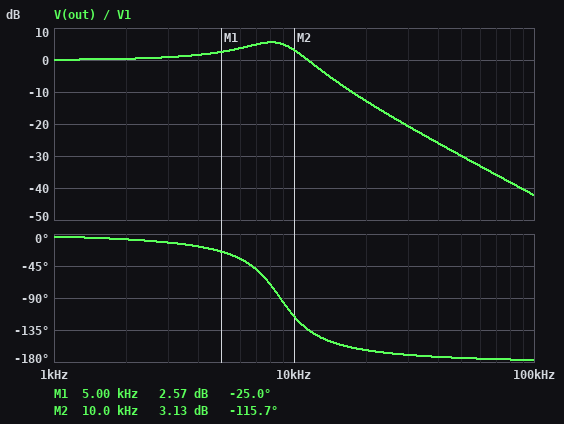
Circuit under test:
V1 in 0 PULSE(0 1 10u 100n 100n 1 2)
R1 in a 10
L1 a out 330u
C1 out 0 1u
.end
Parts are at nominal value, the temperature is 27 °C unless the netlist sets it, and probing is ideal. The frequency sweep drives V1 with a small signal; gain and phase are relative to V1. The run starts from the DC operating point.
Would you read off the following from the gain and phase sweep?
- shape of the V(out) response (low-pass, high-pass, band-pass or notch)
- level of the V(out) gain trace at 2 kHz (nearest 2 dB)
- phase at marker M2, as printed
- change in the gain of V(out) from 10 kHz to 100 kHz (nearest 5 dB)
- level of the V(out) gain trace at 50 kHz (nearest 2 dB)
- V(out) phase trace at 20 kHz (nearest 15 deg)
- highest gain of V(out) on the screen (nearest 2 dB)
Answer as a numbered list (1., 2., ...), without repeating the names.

1. low-pass
2. 0 dB
3. -115.7 deg
4. -45 dB
5. -30 dB
6. -165 deg
7. 6 dB
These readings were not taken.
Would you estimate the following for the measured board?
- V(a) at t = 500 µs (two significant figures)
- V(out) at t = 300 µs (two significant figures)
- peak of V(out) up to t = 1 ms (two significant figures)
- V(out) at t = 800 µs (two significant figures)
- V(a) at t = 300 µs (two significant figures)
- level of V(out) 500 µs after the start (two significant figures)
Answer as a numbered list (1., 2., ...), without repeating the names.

1. 1.0 V
2. 1.0 V
3. 1.4 V
4. 1.0 V
5. 1.0 V
6. 1.0 V
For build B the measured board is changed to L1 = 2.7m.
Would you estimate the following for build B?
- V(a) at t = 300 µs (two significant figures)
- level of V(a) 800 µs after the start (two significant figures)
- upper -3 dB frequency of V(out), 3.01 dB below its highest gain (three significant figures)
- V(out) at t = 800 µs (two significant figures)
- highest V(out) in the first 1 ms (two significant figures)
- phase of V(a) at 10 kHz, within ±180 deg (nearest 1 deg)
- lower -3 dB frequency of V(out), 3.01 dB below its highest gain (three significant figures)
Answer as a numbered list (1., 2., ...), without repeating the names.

1. 1.1 V
2. 980 mV
3. 3.32 kHz
4. 1.2 V
5. 1.7 V
6. 4 deg
7. 2.72 kHz
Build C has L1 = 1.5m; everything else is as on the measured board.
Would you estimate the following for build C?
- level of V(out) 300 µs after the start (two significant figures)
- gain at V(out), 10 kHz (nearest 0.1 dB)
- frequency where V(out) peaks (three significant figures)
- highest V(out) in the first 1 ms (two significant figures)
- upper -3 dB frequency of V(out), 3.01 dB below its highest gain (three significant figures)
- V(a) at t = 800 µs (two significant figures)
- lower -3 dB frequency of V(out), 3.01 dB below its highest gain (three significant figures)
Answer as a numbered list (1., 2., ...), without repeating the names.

1. 800 mV
2. -13.9 dB
3. 4.04 kHz
4. 1.7 V
5. 4.54 kHz
6. 980 mV
7. 3.46 kHz
